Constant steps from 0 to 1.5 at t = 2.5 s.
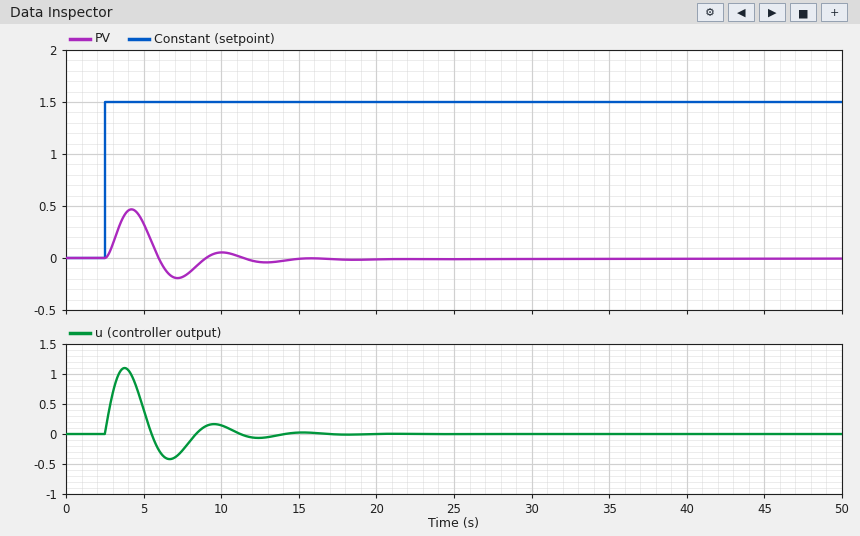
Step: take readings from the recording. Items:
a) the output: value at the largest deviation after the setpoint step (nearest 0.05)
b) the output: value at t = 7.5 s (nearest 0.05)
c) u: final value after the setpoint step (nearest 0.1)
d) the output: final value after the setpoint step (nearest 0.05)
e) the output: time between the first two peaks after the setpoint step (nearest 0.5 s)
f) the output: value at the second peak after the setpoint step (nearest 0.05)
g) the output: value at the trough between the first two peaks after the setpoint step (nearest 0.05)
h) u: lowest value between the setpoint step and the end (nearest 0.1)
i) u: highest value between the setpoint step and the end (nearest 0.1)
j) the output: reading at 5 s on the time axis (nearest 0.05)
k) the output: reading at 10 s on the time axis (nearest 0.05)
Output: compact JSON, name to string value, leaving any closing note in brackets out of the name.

{"the output: value at the largest deviation after the setpoint step": "0.45", "the output: value at t = 7.5 s": "-0.20", "u: final value after the setpoint step": "0.0", "the output: final value after the setpoint step": "0.00", "the output: time between the first two peaks after the setpoint step": "6.0 s", "the output: value at the second peak after the setpoint step": "0.05", "the output: value at the trough between the first two peaks after the setpoint step": "-0.20", "u: lowest value between the setpoint step and the end": "-0.4", "u: highest value between the setpoint step and the end": "1.1", "the output: reading at 5 s on the time axis": "0.35", "the output: reading at 10 s on the time axis": "0.05"}
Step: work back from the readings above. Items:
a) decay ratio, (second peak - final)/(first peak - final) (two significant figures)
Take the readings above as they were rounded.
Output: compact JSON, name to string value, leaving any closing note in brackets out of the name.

{"decay ratio, (second peak - final)/(first peak - final)": "0.11"}
